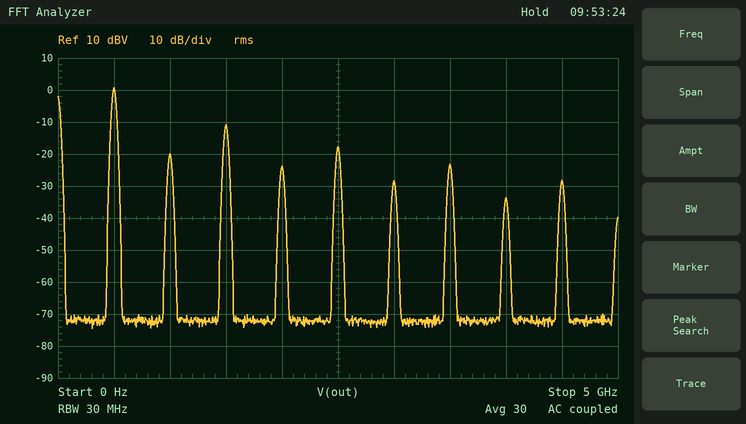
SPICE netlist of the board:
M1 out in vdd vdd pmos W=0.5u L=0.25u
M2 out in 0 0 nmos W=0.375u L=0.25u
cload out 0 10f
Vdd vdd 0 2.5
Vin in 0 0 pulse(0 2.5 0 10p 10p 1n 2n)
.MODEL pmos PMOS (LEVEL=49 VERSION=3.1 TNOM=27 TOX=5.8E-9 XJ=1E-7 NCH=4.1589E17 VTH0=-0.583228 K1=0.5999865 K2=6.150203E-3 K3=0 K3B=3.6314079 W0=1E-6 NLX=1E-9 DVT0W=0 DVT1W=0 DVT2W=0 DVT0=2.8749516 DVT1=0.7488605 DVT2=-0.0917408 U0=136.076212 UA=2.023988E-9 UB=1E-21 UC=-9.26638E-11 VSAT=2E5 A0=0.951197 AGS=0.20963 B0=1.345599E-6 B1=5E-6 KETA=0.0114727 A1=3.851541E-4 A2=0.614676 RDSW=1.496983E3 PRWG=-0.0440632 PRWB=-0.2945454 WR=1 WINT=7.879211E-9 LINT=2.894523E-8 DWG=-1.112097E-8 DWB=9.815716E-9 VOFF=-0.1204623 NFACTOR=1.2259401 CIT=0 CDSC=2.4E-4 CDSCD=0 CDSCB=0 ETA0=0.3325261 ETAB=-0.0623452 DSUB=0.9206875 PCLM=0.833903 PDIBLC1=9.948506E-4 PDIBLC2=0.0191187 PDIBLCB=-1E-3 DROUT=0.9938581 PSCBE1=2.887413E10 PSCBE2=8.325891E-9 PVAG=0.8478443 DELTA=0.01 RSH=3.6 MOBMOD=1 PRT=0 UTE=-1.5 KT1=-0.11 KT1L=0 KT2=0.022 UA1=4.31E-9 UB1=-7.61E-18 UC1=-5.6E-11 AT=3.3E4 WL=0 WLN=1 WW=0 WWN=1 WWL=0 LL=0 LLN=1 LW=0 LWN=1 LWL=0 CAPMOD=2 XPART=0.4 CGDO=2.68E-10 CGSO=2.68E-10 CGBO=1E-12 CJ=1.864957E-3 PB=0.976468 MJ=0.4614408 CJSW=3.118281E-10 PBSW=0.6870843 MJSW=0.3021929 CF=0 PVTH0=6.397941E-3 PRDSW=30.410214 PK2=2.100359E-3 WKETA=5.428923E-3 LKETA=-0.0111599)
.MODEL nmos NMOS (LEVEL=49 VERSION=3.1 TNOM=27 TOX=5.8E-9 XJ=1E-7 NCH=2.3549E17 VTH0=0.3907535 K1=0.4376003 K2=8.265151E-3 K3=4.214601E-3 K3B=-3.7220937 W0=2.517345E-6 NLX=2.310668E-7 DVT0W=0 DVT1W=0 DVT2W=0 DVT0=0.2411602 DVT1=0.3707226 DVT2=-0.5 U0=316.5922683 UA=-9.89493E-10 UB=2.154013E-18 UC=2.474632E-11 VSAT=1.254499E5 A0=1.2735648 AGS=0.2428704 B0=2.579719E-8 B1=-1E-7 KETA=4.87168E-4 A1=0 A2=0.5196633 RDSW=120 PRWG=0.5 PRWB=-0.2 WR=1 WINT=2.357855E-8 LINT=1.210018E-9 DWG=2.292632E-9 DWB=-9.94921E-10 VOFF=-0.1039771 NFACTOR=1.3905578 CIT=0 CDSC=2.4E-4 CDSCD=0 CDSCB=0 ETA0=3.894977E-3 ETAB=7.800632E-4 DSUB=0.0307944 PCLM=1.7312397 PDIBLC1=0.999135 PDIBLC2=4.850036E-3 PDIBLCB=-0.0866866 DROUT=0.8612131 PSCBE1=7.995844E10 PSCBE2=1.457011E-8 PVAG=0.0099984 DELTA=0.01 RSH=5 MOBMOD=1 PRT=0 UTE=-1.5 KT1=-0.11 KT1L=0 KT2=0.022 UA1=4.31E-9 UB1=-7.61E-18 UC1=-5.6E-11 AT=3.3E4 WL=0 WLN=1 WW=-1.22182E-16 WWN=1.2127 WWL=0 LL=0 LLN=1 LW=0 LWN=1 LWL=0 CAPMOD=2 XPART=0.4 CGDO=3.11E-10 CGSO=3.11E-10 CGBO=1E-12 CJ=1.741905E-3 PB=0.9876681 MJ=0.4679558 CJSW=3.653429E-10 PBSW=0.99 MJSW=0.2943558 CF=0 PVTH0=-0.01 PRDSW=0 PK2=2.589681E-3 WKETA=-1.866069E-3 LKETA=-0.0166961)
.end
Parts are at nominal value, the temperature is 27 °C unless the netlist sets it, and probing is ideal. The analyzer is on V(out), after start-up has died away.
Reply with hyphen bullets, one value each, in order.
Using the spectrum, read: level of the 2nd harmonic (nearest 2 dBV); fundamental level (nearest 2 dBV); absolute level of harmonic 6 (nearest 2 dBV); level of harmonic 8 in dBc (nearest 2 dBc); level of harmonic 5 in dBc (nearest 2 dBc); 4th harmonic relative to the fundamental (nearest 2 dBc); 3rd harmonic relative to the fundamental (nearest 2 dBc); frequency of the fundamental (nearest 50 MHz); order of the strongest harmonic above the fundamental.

- -20 dBV
- 0 dBV
- -28 dBV
- -34 dBc
- -18 dBc
- -24 dBc
- -12 dBc
- 500 MHz
- 3
